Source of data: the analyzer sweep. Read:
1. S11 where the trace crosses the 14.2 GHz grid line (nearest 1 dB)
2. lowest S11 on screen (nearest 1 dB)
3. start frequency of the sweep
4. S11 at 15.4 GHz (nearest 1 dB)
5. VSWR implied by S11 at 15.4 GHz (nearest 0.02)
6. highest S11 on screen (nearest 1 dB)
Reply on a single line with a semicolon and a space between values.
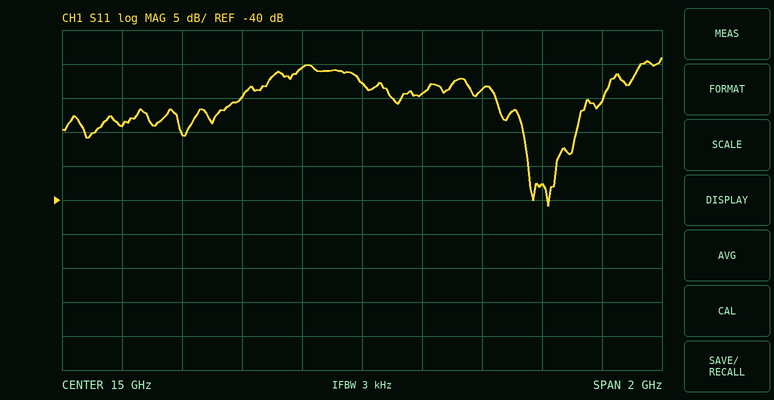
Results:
-29 dB; -41 dB; 14 GHz; -24 dB; 1.14; -19 dB
